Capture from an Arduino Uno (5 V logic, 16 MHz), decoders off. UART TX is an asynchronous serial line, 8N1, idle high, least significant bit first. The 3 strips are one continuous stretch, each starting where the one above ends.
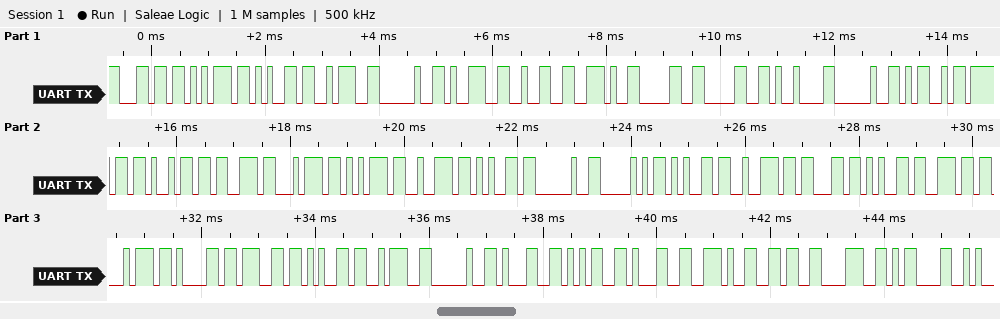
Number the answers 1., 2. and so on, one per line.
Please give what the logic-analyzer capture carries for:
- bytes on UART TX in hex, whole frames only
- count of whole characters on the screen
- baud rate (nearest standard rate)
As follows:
1. 6C 75 65 3A 20 39 32 2E 30 30 09 20 4D 6F 69 73 74 75 72 65 20 50 65 72 63 65 6E 74 61 67 65 3A 20 31 35 31 2E 36 38 0D
2. 40
3. 9600 baud
